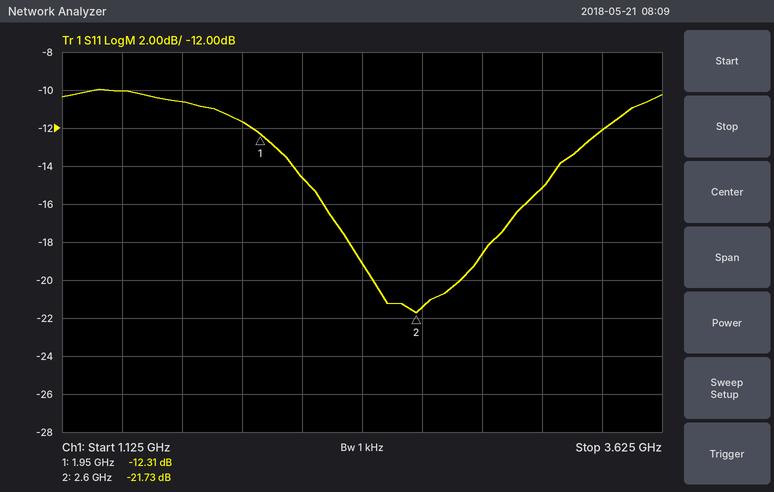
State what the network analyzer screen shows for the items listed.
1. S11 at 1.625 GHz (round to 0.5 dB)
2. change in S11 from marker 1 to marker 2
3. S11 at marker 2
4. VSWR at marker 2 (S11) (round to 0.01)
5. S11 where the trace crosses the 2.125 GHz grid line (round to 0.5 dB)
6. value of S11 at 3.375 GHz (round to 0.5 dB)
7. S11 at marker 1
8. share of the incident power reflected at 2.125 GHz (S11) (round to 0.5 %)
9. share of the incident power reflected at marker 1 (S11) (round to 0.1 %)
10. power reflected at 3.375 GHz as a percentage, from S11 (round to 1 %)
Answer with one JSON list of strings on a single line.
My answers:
["-10.5 dB", "-9.42 dB", "-21.73 dB", "1.18", "-14.5 dB", "-12.0 dB", "-12.31 dB", "3.5 %", "5.9 %", "6 %"]
